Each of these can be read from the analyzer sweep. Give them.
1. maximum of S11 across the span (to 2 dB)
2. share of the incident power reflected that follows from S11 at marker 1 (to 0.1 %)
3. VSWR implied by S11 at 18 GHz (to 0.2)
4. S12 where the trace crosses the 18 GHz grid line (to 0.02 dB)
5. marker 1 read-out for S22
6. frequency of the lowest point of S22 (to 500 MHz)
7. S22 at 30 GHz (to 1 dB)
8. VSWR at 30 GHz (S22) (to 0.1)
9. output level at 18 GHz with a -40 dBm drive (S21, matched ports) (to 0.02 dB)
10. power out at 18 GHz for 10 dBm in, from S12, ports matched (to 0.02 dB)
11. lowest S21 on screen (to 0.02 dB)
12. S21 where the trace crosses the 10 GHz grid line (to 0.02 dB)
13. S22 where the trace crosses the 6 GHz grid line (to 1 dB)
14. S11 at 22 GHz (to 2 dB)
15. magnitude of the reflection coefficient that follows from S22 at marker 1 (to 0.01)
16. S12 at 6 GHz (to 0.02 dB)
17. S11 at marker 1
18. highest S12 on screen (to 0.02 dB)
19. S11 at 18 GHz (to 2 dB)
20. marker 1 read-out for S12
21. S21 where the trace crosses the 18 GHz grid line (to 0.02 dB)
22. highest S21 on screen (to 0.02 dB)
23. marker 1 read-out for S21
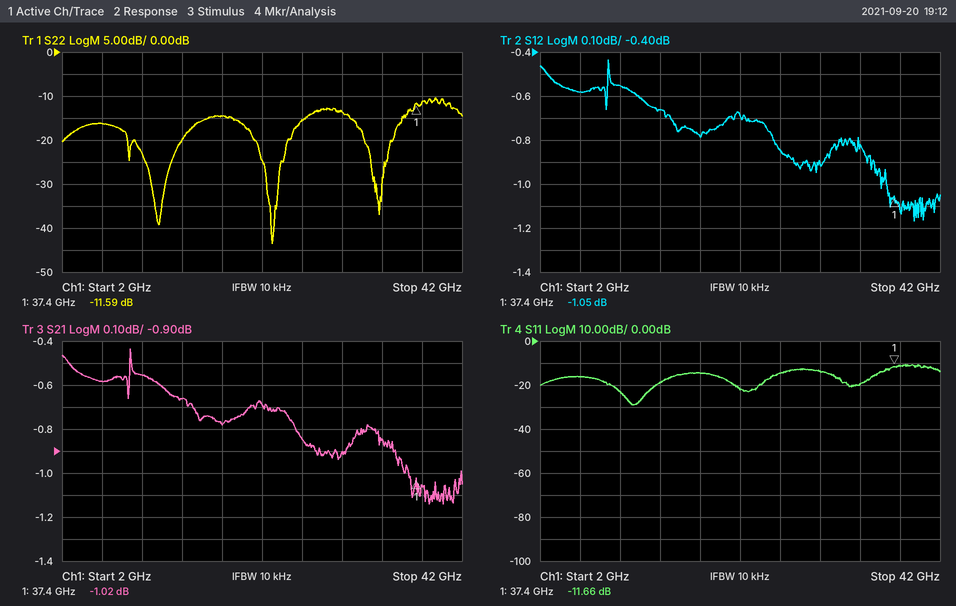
-10 dB
6.8 %
1.4
-0.78 dB
-11.59 dB
23.0 GHz
-14 dB
1.5
-40.78 dBm
9.22 dBm
-1.14 dB
-0.56 dB
-16 dB
-22 dB
0.26
-0.58 dB
-11.66 dB
-0.44 dB
-14 dB
-1.05 dB
-0.78 dB
-0.44 dB
-1.02 dB
